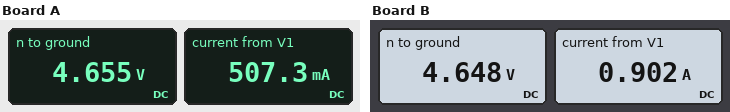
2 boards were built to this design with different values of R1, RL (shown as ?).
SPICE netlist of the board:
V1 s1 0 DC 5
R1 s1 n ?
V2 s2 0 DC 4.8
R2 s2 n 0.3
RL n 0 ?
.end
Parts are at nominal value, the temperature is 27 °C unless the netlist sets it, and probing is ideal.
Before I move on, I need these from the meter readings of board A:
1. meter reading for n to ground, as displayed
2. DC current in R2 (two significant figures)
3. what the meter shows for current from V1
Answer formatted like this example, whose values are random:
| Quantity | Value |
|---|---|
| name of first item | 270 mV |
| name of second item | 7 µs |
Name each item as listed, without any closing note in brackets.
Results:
| Quantity | Value |
|---|---|
| meter reading for n to ground, as displayed | 4.655 V |
| DC current in R2 | 480 mA |
| what the meter shows for current from V1 | 507.3 mA |
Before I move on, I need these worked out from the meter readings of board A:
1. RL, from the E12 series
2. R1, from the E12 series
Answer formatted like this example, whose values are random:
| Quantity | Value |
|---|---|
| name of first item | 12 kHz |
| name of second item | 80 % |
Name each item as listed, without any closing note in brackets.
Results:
| Quantity | Value |
|---|---|
| RL, from the E12 series | 4.7 Ω |
| R1, from the E12 series | 0.68 Ω |
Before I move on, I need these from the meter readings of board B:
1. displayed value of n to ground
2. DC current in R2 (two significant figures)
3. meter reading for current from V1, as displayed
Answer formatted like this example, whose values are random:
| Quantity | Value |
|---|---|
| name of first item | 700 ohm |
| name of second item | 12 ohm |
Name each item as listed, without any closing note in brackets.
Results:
| Quantity | Value |
|---|---|
| displayed value of n to ground | 4.648 V |
| DC current in R2 | 510 mA |
| meter reading for current from V1, as displayed | 0.902 A |
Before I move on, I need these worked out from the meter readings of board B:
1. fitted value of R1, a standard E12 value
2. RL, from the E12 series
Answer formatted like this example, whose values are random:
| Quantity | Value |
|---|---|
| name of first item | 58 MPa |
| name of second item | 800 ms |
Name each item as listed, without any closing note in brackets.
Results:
| Quantity | Value |
|---|---|
| fitted value of R1, a standard E12 value | 0.39 Ω |
| RL, from the E12 series | 3.3 Ω |
